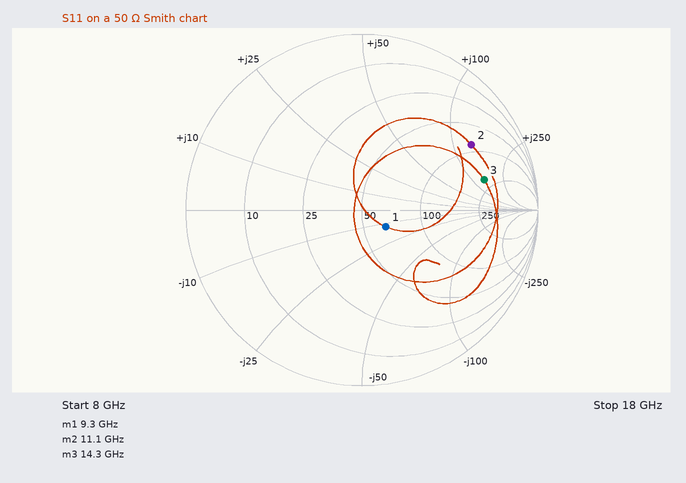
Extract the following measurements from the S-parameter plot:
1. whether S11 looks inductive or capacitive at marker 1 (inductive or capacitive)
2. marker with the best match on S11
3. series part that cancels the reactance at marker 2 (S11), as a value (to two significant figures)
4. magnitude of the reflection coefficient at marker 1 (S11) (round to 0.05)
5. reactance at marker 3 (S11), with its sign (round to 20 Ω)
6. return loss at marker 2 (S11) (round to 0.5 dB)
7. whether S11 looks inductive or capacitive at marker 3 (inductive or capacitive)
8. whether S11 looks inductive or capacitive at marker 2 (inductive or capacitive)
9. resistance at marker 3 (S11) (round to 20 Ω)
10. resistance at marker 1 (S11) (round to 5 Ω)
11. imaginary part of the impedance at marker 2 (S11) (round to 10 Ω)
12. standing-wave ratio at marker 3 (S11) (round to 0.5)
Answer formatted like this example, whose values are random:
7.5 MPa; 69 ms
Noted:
capacitive; marker 1; 110 fF; 0.15; +140 Ω; 3.0 dB; inductive; inductive; 200 Ω; 65 Ω; +130 Ω; 6.0
